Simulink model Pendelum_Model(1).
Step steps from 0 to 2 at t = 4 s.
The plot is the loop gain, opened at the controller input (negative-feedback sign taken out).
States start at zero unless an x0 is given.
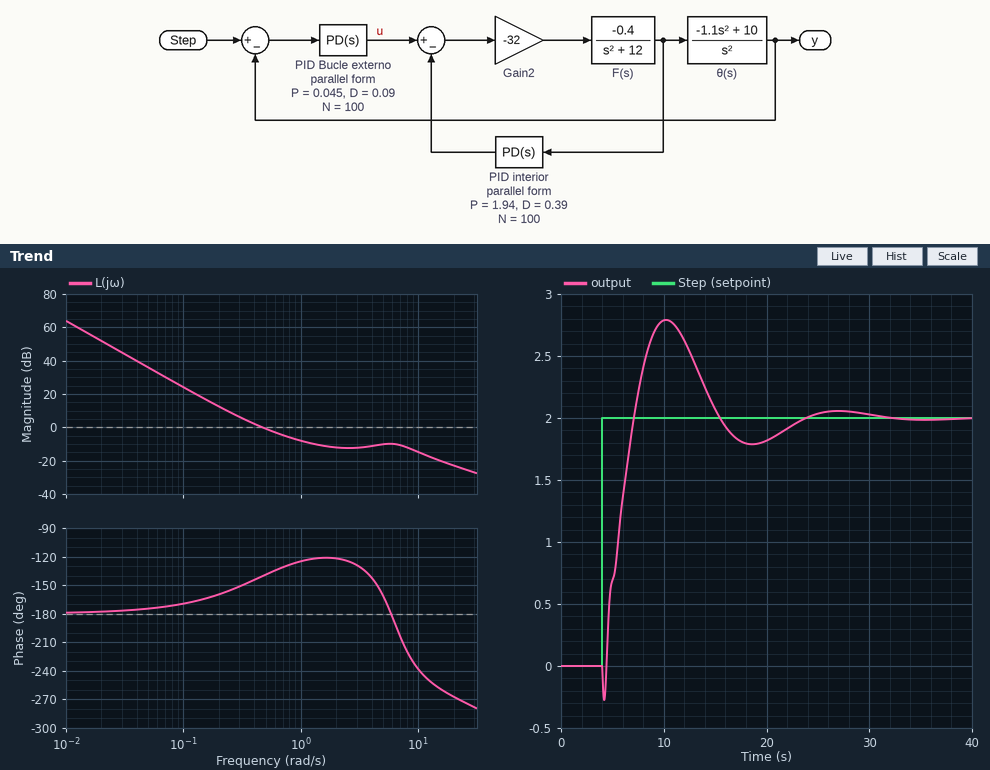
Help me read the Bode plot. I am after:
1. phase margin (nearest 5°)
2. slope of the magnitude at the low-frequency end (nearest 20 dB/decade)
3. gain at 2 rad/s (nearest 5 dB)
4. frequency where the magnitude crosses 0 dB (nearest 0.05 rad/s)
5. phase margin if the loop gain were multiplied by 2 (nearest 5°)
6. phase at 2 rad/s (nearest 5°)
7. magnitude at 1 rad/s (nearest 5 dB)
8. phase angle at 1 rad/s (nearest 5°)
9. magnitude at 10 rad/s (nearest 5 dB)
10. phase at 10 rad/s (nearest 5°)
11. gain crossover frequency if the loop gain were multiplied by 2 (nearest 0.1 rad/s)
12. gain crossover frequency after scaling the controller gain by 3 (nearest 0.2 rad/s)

40°
-40 dB/decade
-10 dB
0.45 rad/s
50°
-120°
-10 dB
-125°
-15 dB
-240°
0.8 rad/s
1.2 rad/s
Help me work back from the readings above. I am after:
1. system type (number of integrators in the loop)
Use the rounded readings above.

2
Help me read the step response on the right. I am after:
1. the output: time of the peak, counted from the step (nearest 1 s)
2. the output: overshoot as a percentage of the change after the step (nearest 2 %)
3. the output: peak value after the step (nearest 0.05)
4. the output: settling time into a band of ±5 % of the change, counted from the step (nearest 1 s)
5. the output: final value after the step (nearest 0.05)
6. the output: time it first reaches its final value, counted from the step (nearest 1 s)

6 s
40 %
2.80
18 s
2.00
3 s
